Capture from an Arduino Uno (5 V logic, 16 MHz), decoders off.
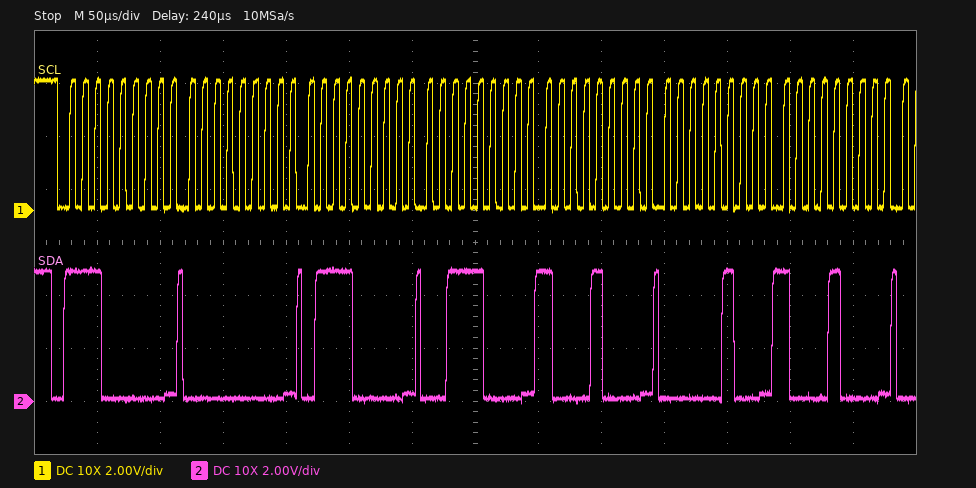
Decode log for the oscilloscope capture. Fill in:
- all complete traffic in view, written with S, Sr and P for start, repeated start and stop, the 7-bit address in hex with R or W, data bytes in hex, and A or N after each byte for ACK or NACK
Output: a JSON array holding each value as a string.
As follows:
["S 70W A 00 A 70 A 38 A 88 A 04 A 88 A"]
